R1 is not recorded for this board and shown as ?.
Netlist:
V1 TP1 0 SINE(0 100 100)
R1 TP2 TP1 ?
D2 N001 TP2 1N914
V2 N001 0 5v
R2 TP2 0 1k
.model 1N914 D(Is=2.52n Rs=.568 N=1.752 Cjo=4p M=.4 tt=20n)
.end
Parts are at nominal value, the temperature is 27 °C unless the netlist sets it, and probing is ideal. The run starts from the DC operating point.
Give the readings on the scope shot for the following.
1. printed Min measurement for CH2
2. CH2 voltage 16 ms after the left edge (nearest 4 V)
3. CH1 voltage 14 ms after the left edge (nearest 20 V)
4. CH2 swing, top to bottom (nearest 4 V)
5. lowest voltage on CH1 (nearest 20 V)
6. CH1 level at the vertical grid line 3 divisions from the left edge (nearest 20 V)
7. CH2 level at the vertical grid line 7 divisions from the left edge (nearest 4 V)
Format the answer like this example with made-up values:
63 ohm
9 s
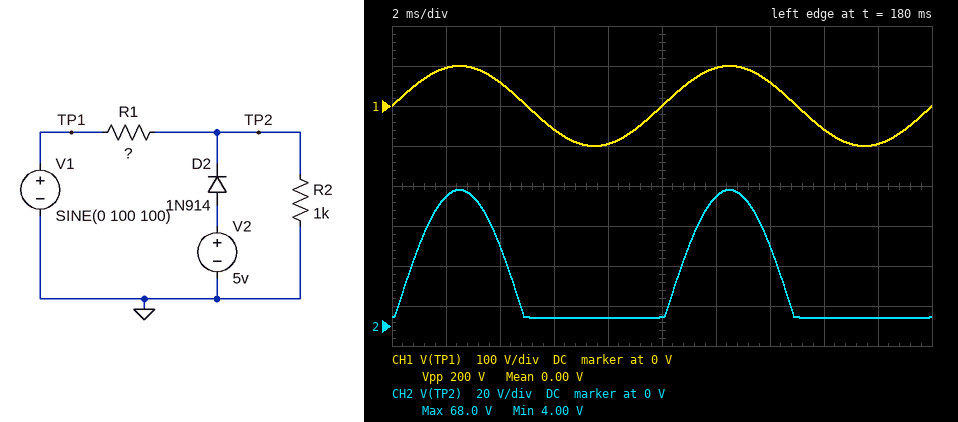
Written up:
4.00 V
4 V
60 V
64 V
-100 V
-60 V
40 V
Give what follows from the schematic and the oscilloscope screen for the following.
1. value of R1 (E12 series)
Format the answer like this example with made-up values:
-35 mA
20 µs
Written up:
470 Ω
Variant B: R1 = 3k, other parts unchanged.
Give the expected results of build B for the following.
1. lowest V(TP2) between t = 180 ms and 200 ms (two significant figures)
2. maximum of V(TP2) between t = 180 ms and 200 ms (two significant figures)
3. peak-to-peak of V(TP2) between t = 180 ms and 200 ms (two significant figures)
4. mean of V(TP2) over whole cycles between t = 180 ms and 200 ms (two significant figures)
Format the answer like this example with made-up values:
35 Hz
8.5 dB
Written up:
4.2 V
25 V
21 V
10 V
